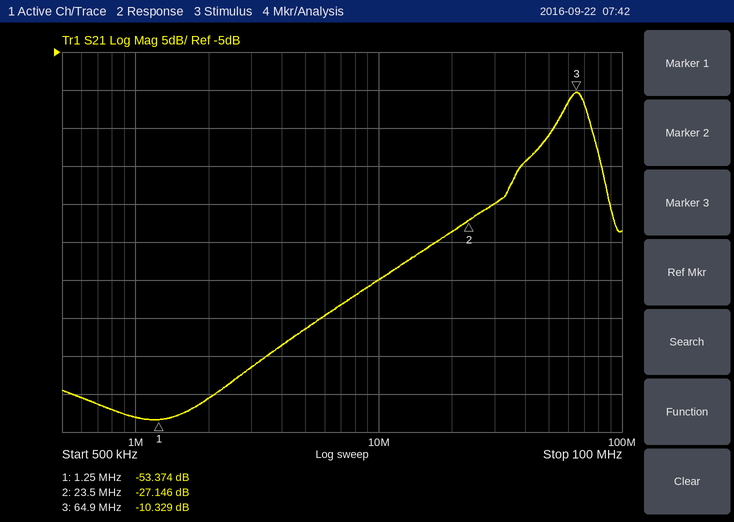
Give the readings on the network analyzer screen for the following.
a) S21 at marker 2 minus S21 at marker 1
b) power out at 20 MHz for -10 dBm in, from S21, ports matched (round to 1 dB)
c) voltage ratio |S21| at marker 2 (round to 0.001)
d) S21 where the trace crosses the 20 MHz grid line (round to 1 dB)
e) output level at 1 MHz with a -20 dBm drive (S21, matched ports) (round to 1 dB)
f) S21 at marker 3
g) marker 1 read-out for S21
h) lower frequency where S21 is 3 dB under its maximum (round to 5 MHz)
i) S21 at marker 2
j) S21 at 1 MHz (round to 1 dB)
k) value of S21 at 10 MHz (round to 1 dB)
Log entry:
26.228 dB
-39 dBm
0.044
-29 dB
-73 dBm
-10.329 dB
-53.374 dB
55 MHz
-27.146 dB
-53 dB
-35 dB
